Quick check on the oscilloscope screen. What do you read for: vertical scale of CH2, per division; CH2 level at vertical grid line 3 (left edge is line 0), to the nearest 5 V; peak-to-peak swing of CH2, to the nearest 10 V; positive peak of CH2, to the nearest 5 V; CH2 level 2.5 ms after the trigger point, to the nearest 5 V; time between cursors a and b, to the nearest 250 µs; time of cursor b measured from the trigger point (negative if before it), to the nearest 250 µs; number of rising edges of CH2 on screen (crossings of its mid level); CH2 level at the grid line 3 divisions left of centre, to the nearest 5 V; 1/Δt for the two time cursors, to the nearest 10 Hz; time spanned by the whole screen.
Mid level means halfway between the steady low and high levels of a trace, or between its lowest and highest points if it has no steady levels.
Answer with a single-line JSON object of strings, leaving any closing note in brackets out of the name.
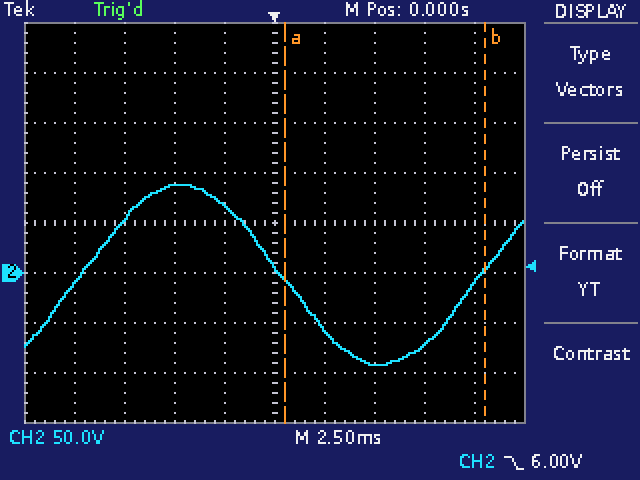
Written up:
{"vertical scale of CH2, per division": "50 V", "CH2 level at vertical grid line 3 (left edge is line 0), to the nearest 5 V": "90 V", "peak-to-peak swing of CH2, to the nearest 10 V": "180 V", "positive peak of CH2, to the nearest 5 V": "90 V", "CH2 level 2.5 ms after the trigger point, to the nearest 5 V": "-55 V", "time between cursors a and b, to the nearest 250 µs": "10.00 ms", "time of cursor b measured from the trigger point (negative if before it), to the nearest 250 µs": "+10.50 ms", "number of rising edges of CH2 on screen": "2", "CH2 level at the grid line 3 divisions left of centre, to the nearest 5 V": "55 V", "1/Δt for the two time cursors, to the nearest 10 Hz": "100 Hz", "time spanned by the whole screen": "25 ms"}
